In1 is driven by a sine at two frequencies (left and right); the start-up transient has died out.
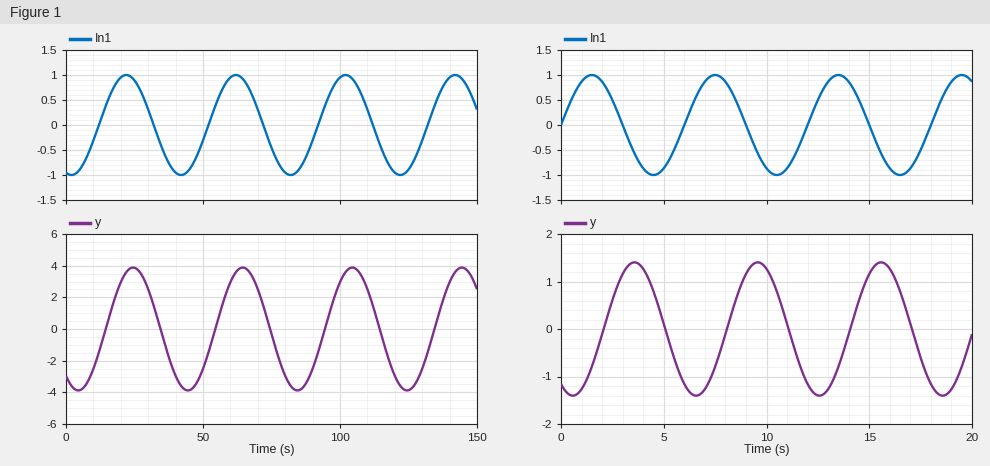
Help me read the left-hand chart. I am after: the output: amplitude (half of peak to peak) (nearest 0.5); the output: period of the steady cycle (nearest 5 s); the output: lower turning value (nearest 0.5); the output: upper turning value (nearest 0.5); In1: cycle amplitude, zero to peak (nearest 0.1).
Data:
4.0
40 s
-4.0
4.0
1.0
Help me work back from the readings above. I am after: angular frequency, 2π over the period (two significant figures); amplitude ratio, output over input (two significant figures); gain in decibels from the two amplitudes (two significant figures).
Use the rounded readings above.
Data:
0.16 rad/s
4.0
12 dB
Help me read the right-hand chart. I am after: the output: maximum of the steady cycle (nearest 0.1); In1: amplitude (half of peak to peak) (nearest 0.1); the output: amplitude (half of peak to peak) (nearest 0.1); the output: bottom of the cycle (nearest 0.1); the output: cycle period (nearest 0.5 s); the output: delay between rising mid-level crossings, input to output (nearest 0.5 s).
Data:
1.4
1.0
1.4
-1.4
6.0 s
2.0 s
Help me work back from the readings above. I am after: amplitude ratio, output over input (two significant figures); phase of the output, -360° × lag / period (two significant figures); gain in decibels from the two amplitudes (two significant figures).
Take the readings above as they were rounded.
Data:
1.4
-120°
2.9 dB
